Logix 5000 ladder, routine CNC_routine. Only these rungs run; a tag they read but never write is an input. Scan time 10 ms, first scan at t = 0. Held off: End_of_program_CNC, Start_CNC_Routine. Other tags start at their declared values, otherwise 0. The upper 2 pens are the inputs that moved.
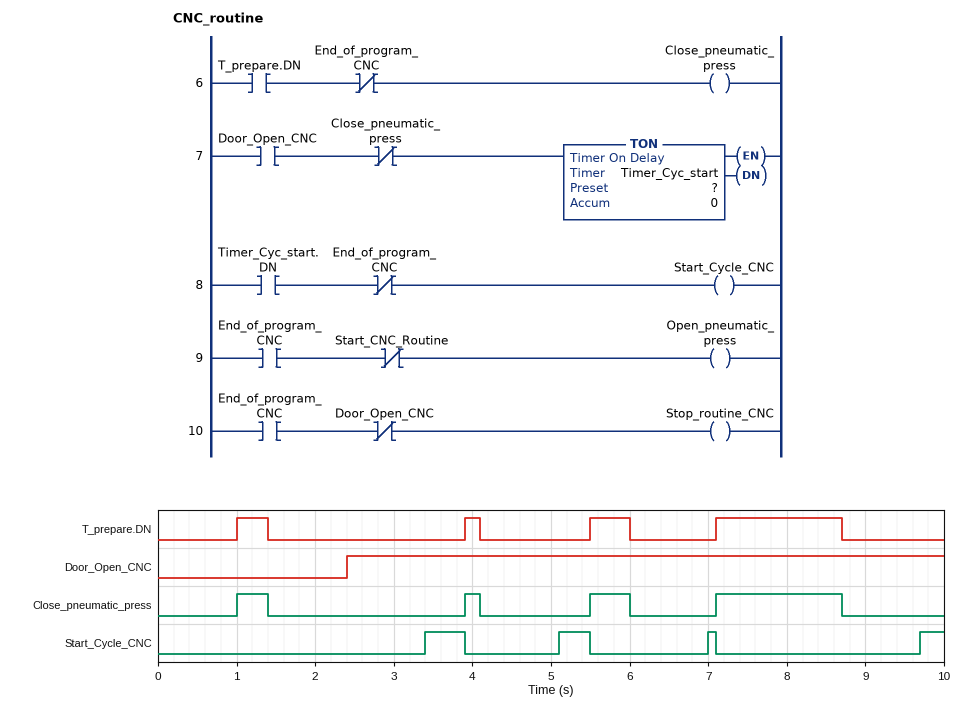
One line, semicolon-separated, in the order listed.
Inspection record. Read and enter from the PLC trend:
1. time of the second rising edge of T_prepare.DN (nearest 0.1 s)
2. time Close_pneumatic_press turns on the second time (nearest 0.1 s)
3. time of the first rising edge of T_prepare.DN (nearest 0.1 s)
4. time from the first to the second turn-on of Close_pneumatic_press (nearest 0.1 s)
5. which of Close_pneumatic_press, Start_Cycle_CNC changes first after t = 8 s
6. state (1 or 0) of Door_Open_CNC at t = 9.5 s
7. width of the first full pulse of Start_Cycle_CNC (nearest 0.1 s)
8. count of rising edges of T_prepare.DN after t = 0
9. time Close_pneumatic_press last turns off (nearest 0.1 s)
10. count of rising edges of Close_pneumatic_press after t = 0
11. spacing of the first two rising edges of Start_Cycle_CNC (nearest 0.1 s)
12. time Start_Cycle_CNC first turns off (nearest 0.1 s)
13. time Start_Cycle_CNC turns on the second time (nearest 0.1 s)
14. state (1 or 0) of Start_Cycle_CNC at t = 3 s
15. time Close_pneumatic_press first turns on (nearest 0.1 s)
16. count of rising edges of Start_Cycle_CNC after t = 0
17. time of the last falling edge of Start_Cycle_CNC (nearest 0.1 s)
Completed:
3.9 s; 3.9 s; 1.0 s; 2.9 s; Close_pneumatic_press; 1; 0.5 s; 4; 8.7 s; 4; 1.7 s; 3.9 s; 5.1 s; 0; 1.0 s; 4; 7.1 s
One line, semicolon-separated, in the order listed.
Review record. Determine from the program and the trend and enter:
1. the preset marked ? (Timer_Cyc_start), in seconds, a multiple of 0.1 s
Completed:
1.0 s
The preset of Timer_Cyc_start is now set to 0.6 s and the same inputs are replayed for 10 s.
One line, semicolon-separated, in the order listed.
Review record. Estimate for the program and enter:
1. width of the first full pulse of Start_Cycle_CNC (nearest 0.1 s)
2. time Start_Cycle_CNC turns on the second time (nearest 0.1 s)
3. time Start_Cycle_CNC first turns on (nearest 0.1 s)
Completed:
0.9 s; 4.7 s; 3.0 s
